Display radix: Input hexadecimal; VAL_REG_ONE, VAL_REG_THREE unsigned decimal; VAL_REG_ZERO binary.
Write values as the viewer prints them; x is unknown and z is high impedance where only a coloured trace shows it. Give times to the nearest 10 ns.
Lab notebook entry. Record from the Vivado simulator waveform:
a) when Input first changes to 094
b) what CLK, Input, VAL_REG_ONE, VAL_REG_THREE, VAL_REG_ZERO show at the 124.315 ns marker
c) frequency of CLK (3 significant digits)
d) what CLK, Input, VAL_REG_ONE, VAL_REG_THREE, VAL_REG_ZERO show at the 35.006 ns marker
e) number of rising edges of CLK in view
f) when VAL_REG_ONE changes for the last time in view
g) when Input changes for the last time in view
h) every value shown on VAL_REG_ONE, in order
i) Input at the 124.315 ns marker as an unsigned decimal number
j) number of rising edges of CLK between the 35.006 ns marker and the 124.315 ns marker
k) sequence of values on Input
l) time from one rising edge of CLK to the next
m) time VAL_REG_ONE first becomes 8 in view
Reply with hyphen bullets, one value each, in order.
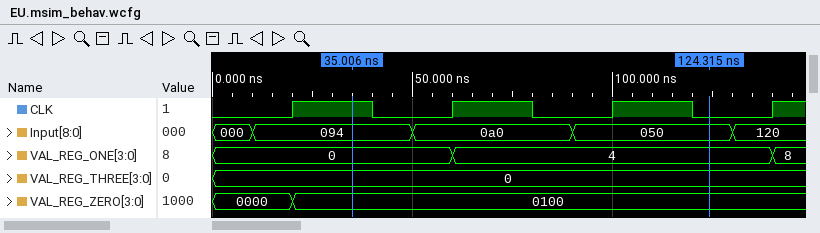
- 10 ns
- CLK=0, Input=050, VAL_REG_ONE=4, VAL_REG_THREE=0, VAL_REG_ZERO=0100
- 25.0 MHz
- CLK=1, Input=094, VAL_REG_ONE=0, VAL_REG_THREE=0, VAL_REG_ZERO=0100
- 4
- 140 ns
- 130 ns
- 0, 4, 8
- 80
- 2
- 000, 094, 0a0, 050, 120
- 40 ns
- 140 ns
